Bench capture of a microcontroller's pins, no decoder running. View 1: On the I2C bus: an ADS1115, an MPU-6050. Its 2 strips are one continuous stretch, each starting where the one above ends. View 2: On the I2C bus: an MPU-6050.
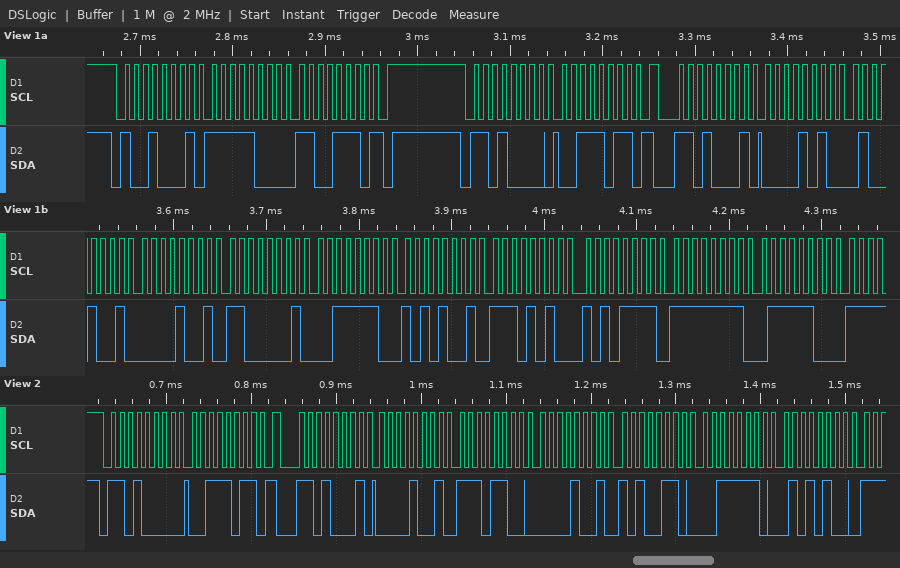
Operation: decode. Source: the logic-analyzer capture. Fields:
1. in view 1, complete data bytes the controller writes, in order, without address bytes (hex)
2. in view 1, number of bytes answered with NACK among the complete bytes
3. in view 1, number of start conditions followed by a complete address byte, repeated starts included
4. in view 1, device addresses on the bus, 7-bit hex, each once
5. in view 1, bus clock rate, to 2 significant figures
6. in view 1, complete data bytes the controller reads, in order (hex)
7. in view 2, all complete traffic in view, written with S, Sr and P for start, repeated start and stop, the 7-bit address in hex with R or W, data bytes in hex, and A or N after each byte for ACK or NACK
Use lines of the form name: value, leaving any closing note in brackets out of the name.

in view 1, complete data bytes the controller writes, in order, without address bytes: 3B
in view 1, number of bytes answered with NACK among the complete bytes: 1
in view 1, number of start conditions followed by a complete address byte, repeated starts included: 3
in view 1, device addresses on the bus, 7-bit hex, each once: 0x48 0x68
in view 1, bus clock rate, to 2 significant figures: 100 kHz
in view 1, complete data bytes the controller reads, in order: F8 CE 0A 49 09 C1 3E A9 EA AF FF 7C
in view 2, all complete traffic in view, written with S, Sr and P for start, repeated start and stop, the 7-bit address in hex with R or W, data bytes in hex, and A or N after each byte for ACK or NACK: S 68W A 3B A Sr 68R A 09 A EC A 09 A A6 A 3E A 54 A
